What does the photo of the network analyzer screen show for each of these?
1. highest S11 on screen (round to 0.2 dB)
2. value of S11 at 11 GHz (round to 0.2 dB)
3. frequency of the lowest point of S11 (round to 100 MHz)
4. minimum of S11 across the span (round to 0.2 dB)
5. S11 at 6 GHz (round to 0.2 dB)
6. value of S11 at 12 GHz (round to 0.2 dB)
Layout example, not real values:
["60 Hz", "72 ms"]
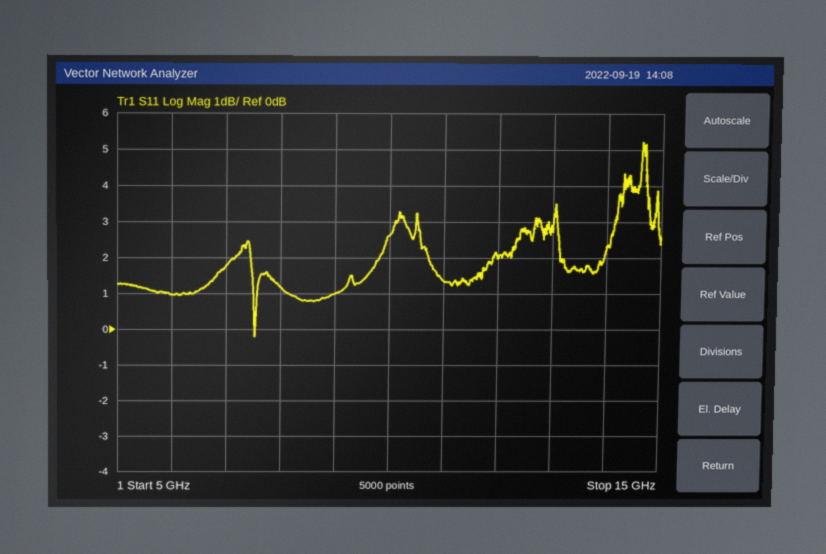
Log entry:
["5.2 dB", "1.4 dB", "7.5 GHz", "-0.2 dB", "1.0 dB", "2.0 dB"]
